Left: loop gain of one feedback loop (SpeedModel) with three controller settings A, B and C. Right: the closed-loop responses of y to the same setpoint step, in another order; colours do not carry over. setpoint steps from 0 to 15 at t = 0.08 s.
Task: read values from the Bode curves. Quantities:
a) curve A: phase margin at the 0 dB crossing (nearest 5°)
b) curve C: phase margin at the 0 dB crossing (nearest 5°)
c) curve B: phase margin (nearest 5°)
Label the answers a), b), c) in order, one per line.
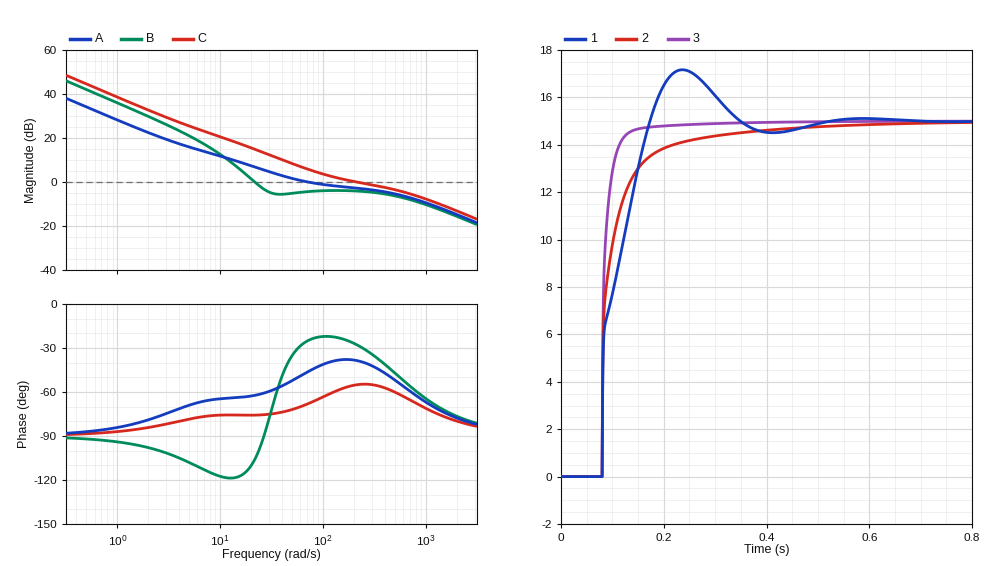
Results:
a) 135°
b) 125°
c) 75°
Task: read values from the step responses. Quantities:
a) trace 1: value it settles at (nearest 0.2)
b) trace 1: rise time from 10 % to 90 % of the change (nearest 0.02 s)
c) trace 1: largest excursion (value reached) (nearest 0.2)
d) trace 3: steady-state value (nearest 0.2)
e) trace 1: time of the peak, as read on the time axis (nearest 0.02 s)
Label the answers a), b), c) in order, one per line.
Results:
a) 15.0
b) 0.08 s
c) 17.2
d) 15.0
e) 0.24 s
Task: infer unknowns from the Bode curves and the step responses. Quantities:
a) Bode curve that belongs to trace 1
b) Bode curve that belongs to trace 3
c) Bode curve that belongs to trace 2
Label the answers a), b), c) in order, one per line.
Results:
a) B
b) C
c) A
